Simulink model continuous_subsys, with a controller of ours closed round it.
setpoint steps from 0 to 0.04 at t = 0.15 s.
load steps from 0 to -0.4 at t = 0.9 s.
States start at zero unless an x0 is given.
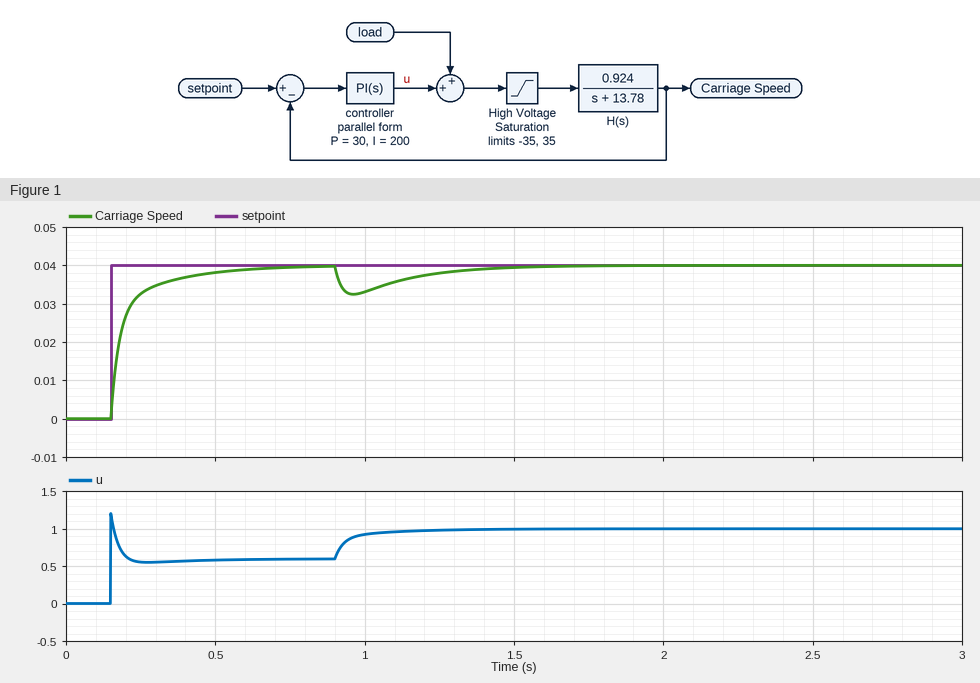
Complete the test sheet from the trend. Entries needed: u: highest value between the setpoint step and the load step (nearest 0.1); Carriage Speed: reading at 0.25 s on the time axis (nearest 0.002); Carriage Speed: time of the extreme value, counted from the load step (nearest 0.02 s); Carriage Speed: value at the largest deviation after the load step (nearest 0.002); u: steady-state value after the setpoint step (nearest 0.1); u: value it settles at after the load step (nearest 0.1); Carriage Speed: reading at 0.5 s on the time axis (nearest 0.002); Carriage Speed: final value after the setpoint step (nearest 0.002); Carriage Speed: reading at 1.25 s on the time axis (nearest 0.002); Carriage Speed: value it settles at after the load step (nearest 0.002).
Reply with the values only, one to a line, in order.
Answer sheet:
1.2
0.032
0.06 s
0.032
0.6
1.0
0.038
0.040
0.038
0.040
